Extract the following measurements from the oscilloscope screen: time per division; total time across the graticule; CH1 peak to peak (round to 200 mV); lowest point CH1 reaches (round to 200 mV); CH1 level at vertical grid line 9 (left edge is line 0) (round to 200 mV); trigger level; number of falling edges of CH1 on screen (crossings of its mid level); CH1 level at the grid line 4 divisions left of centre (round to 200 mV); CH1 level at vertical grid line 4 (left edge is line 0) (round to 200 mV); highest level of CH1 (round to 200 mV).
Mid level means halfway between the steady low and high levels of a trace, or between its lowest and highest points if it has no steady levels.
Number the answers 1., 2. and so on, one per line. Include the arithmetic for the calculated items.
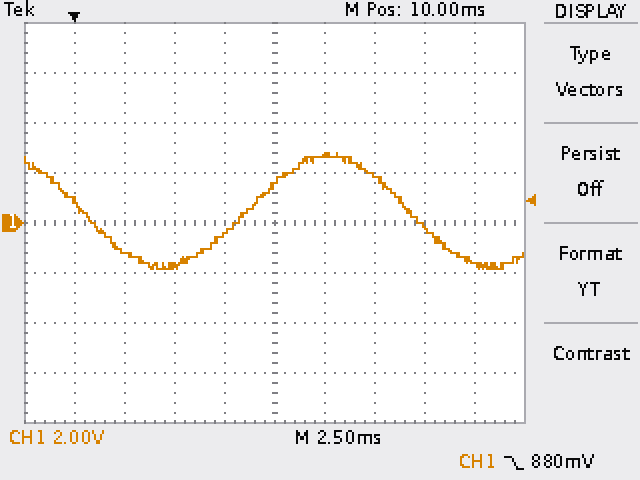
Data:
1. 2.5 ms
2. 25 ms
3. 2.8 V − (-1.8 V) = 4.6 V
4. -1.8 V
5. -1.6 V
6. 880 mV
7. 2
8. 800 mV
9. -400 mV
10. 2.8 V
